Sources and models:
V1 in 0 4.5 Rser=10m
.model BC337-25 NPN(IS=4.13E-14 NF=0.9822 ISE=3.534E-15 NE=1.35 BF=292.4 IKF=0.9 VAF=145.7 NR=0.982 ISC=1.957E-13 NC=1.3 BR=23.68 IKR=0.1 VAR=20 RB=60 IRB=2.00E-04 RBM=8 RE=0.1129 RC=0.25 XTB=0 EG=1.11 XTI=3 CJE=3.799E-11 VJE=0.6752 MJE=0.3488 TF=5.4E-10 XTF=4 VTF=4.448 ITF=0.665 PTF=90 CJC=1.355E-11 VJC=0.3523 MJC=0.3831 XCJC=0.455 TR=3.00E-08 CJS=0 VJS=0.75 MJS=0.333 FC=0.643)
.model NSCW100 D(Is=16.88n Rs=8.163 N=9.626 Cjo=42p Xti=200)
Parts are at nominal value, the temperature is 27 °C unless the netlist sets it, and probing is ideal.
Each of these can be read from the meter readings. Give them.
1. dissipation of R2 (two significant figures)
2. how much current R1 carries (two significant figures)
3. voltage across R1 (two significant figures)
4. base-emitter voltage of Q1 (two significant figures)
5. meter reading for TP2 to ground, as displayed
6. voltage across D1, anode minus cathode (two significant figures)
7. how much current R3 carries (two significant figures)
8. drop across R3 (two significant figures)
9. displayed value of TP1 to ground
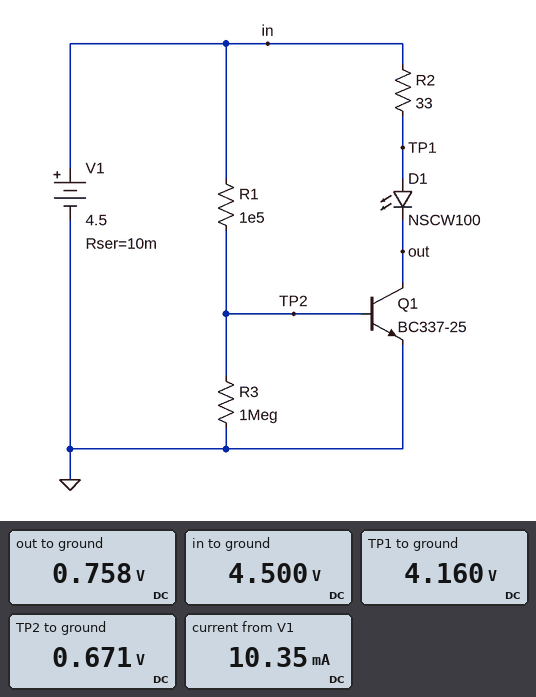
3.5 mW
38 µA
3.8 V
670 mV
0.671 V
3.4 V
670 nA
670 mV
4.160 V
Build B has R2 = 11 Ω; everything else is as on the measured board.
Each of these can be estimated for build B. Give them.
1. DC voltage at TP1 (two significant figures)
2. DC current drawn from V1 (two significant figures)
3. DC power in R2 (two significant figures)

4.4 V
10 mA
1.2 mW
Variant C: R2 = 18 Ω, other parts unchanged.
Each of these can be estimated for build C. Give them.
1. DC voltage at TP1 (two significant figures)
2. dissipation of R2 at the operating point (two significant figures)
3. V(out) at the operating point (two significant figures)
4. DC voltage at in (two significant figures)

4.3 V
1.9 mW
910 mV
4.5 V
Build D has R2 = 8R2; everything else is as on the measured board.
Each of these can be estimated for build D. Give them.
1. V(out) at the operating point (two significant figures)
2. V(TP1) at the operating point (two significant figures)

1.0 V
4.4 V
